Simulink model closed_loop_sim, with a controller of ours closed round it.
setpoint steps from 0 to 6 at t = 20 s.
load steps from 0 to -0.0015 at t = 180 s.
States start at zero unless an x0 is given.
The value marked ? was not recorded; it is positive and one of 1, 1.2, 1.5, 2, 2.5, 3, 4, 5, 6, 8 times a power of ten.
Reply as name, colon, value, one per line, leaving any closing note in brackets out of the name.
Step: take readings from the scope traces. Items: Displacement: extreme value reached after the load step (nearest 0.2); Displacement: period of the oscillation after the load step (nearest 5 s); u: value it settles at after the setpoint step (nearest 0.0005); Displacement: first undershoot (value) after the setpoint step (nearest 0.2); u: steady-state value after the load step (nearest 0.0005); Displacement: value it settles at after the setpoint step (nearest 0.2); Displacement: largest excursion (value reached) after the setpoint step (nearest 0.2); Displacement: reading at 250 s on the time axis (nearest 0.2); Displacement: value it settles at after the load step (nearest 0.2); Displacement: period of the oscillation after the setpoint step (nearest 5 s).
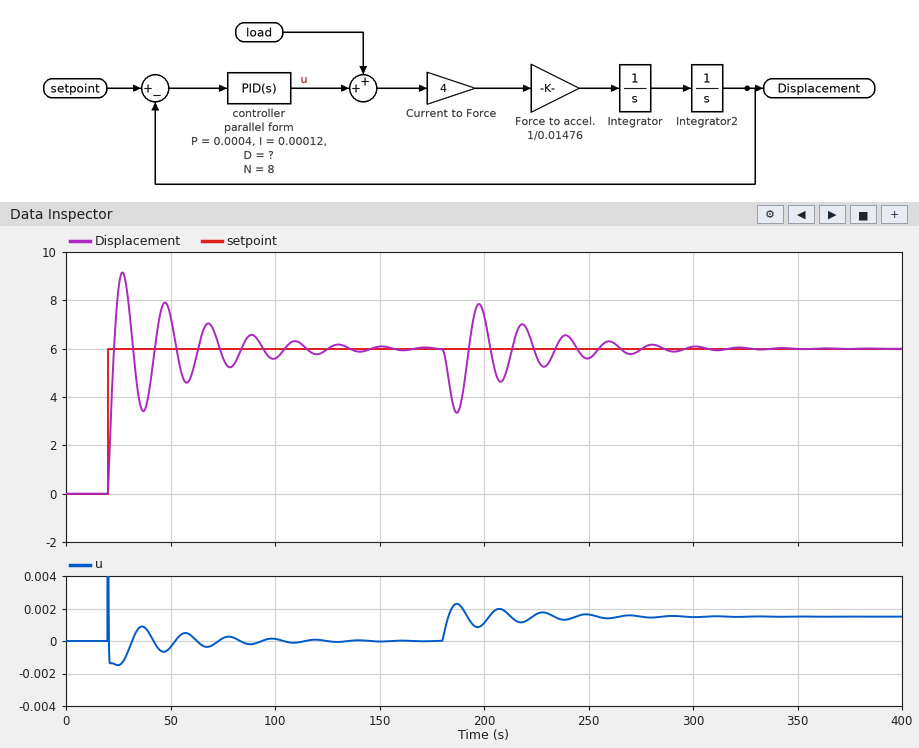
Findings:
Displacement: extreme value reached after the load step: 3.4
Displacement: period of the oscillation after the load step: 20 s
u: value it settles at after the setpoint step: 0.0000
Displacement: first undershoot (value) after the setpoint step: 3.4
u: steady-state value after the load step: 0.0015
Displacement: value it settles at after the setpoint step: 6.0
Displacement: largest excursion (value reached) after the setpoint step: 9.2
Displacement: reading at 250 s on the time axis: 5.6
Displacement: value it settles at after the load step: 6.0
Displacement: period of the oscillation after the setpoint step: 20 s
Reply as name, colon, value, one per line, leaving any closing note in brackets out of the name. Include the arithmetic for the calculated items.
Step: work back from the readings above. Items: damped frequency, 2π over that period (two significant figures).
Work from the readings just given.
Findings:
damped frequency, 2π over that period: 2π / 20 = 0.31 rad/s
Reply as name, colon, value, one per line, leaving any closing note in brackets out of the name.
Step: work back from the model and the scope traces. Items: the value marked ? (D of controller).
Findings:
the value marked ?: 0.0015
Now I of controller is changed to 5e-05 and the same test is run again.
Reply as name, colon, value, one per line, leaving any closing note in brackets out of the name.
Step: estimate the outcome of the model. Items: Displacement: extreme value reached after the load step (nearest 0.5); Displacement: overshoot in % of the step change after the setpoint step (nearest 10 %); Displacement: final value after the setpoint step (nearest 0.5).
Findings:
Displacement: extreme value reached after the load step: 3.0
Displacement: overshoot in % of the step change after the setpoint step: 40 %
Displacement: final value after the setpoint step: 6.0
